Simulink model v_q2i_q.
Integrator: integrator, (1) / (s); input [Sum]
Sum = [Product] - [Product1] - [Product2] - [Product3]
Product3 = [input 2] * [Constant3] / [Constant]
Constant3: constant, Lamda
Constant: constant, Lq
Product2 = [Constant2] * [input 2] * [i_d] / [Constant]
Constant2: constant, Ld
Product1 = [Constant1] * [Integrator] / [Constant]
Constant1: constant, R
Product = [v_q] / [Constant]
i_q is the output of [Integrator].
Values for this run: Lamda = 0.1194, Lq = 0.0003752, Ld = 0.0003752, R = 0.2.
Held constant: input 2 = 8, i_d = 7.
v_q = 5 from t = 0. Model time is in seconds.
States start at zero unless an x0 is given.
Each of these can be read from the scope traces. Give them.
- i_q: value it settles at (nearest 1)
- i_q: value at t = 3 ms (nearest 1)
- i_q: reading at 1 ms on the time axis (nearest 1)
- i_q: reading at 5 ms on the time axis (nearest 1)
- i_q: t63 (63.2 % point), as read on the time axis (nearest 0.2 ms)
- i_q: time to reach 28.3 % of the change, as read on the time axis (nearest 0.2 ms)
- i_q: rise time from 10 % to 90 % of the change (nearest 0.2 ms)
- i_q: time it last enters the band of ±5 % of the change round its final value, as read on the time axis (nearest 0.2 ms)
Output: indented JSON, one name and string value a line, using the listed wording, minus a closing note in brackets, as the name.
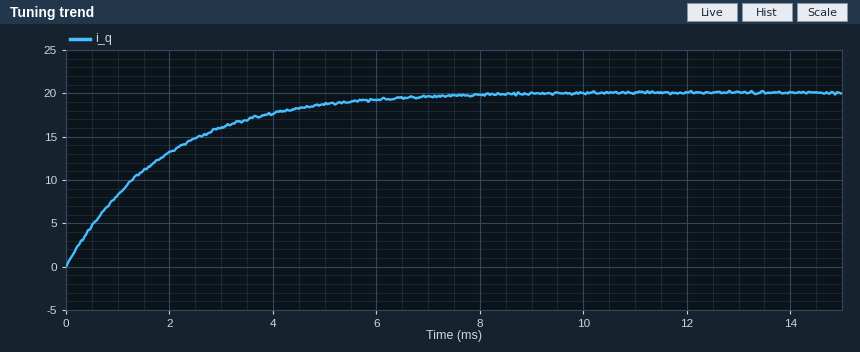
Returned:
{
  "i_q: value it settles at": "20",
  "i_q: value at t = 3 ms": "16",
  "i_q: reading at 1 ms on the time axis": "8",
  "i_q: reading at 5 ms on the time axis": "19",
  "i_q: t63 (63.2 % point), as read on the time axis": "1.8 ms",
  "i_q: time to reach 28.3 % of the change, as read on the time axis": "0.6 ms",
  "i_q: rise time from 10 % to 90 % of the change": "4.2 ms",
  "i_q: time it last enters the band of ±5 % of the change round its final value, as read on the time axis": "5.6 ms"
}
